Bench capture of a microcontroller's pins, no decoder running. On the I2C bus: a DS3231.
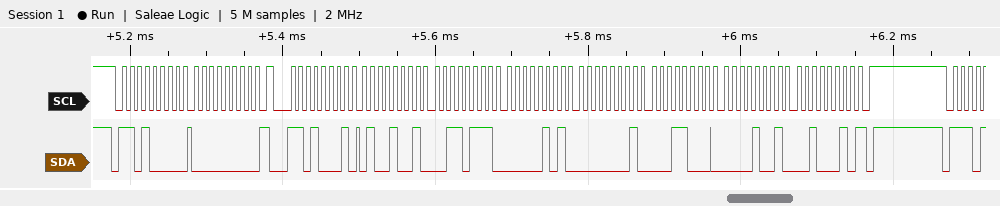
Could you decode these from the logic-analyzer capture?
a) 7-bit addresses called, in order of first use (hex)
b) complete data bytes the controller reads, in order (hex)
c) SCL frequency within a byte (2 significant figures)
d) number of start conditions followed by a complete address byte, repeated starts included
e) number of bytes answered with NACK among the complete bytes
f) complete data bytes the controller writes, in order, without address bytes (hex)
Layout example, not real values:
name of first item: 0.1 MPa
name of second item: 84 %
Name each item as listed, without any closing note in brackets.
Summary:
7-bit addresses called, in order of first use: 0x68
complete data bytes the controller reads, in order: 49 37 05 01 18 09 22
SCL frequency within a byte: 100 kHz
number of start conditions followed by a complete address byte, repeated starts included: 2
number of bytes answered with NACK among the complete bytes: 1
complete data bytes the controller writes, in order, without address bytes: 00
